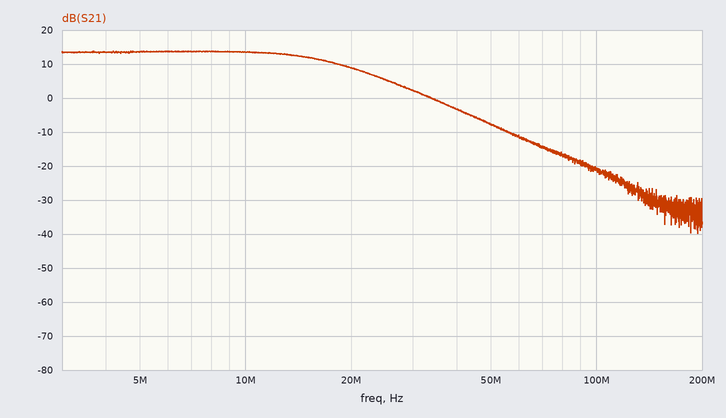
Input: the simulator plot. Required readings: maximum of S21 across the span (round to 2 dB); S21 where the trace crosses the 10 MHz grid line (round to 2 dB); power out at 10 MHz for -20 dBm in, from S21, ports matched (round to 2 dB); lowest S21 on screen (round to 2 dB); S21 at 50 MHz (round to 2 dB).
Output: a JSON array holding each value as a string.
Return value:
["14 dB", "14 dB", "-6 dBm", "-40 dB", "-8 dB"]
